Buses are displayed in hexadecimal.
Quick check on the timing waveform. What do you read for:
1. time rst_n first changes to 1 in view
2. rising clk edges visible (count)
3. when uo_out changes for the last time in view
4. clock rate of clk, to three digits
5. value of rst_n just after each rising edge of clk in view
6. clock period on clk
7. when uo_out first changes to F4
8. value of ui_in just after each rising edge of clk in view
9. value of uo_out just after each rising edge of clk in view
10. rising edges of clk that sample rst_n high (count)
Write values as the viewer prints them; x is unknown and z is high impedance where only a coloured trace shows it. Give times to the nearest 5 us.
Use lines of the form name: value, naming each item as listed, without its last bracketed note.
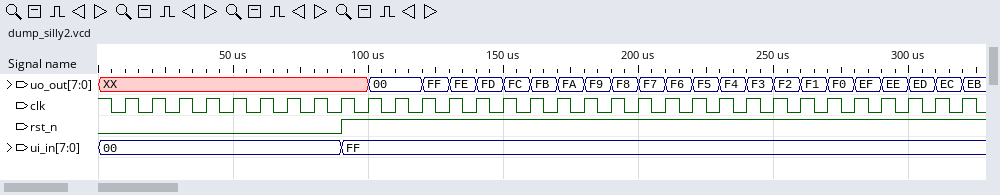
time rst_n first changes to 1 in view: 90 us
rising clk edges visible: 32
when uo_out changes for the last time in view: 320 us
clock rate of clk, to three digits: 100 kHz
value of rst_n just after each rising edge of clk in view: 0 0 0 0 0 0 0 0 1 1 1 1 1 1 1 1 1 1 1 1 1 1 1 1 1 1 1 1 1 1 1 1
clock period on clk: 10 us
when uo_out first changes to F4: 230 us
value of ui_in just after each rising edge of clk in view: 00, 00, 00, 00, 00, 00, 00, 00, FF, FF, FF, FF, FF, FF, FF, FF, FF, FF, FF, FF, FF, FF, FF, FF, FF, FF, FF, FF, FF, FF, FF, FF
value of uo_out just after each rising edge of clk in view: XX, XX, XX, XX, XX, XX, XX, XX, XX, 00, 00, FF, FE, FD, FC, FB, FA, F9, F8, F7, F6, F5, F4, F3, F2, F1, F0, EF, EE, ED, EC, EB
rising edges of clk that sample rst_n high: 23
